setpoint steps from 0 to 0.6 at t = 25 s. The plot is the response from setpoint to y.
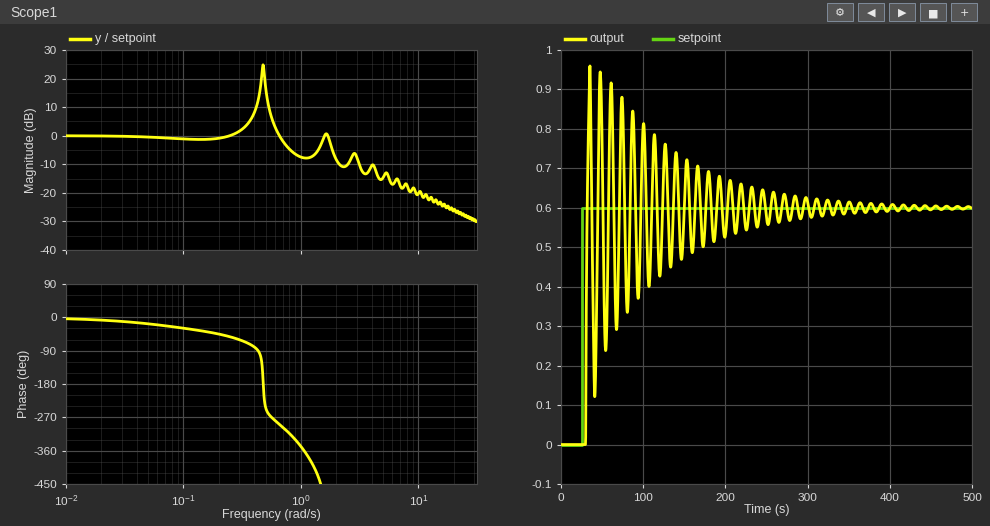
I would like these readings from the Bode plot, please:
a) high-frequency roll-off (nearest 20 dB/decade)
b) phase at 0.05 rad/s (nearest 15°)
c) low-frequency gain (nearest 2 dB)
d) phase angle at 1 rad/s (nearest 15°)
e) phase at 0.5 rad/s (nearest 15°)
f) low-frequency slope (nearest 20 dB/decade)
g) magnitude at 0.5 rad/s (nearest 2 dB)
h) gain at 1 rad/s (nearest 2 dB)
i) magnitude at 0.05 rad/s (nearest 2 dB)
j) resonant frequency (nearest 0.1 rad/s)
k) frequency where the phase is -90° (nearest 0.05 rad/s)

-20 dB/decade
-15°
0 dB
-345°
-240°
0 dB/decade
18 dB
-8 dB
0 dB
0.5 rad/s
0.45 rad/s
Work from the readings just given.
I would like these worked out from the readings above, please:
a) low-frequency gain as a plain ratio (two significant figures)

1.0
